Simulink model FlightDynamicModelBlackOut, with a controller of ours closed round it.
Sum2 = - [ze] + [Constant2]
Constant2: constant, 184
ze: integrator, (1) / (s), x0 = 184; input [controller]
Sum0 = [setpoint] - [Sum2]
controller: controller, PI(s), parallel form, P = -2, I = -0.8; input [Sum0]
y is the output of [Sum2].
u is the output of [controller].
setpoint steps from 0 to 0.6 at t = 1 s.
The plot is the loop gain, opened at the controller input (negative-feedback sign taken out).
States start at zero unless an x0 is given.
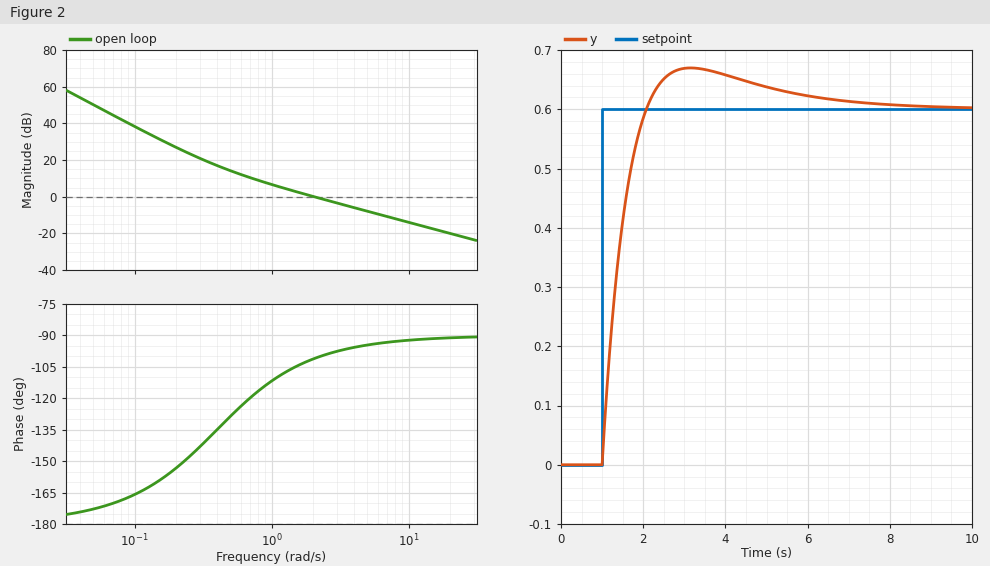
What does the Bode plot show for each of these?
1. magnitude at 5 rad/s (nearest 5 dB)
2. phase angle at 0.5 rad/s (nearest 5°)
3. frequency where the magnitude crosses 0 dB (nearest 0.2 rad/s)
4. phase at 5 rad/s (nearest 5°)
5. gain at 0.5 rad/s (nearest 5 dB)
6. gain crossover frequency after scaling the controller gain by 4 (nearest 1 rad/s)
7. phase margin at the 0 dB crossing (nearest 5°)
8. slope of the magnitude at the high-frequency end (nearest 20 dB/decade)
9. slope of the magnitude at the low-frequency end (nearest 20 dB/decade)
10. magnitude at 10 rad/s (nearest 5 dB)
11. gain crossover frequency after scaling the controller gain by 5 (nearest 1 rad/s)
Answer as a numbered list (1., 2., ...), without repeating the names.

1. -10 dB
2. -130°
3. 2.0 rad/s
4. -95°
5. 15 dB
6. 8 rad/s
7. 80°
8. -20 dB/decade
9. -40 dB/decade
10. -15 dB
11. 10 rad/s
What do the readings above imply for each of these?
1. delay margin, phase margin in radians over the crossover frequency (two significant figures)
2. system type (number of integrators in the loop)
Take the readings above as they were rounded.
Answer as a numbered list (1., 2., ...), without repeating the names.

1. 0.70 s
2. 2
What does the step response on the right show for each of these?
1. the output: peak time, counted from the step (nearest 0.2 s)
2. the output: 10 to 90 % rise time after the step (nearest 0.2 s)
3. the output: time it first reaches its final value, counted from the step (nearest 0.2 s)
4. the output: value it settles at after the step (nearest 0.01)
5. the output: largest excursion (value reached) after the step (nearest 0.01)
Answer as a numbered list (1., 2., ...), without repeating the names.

1. 2.2 s
2. 0.8 s
3. 1.0 s
4. 0.60
5. 0.67
